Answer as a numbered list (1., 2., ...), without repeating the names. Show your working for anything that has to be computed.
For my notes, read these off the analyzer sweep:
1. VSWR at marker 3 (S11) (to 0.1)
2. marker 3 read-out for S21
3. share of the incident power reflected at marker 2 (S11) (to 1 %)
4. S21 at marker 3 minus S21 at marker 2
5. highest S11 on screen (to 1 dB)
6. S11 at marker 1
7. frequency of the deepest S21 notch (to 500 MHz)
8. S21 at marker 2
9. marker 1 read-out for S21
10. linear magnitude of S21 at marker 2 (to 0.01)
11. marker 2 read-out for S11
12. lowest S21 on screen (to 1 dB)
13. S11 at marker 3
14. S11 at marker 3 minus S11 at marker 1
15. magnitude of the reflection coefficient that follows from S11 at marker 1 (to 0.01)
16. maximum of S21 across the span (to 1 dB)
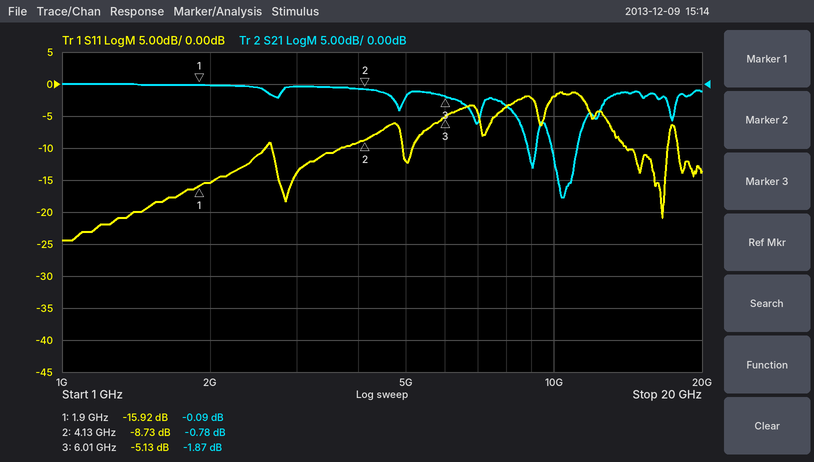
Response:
1. (1 + 0.5540)/(1 − 0.5540) ≈ 3.5
2. -1.87 dB
3. 10^(-8.73/10) ≈ 13 %
4. -1.87 − (-0.78) = -1.09 dB
5. -1 dB
6. -15.92 dB
7. 10.5 GHz
8. -0.78 dB
9. -0.09 dB
10. 10^(-0.78/20) ≈ 0.91
11. -8.73 dB
12. -18 dB
13. -5.13 dB
14. -5.13 − (-15.92) = 10.79 dB
15. 10^(-15.92/20) ≈ 0.16
16. 0 dB
